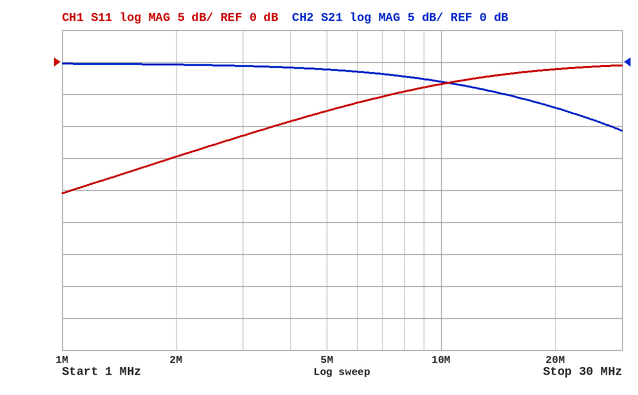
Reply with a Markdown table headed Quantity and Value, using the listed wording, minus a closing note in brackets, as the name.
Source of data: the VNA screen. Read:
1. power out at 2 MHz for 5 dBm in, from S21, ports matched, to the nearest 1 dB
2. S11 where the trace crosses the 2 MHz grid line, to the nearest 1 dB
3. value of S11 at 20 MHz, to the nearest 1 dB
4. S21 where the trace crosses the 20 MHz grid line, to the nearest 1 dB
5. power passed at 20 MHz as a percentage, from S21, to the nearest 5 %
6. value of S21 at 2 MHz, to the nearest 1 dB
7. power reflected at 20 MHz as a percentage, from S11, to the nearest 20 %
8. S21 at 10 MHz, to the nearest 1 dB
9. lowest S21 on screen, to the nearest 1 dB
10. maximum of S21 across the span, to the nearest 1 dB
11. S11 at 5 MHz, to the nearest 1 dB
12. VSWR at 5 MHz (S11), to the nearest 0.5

| Quantity | Value |
|---|---|
| power out at 2 MHz for 5 dBm in, from S21, ports matched, to the nearest 1 dB | 5 dBm |
| S11 where the trace crosses the 2 MHz grid line, to the nearest 1 dB | -15 dB |
| value of S11 at 20 MHz, to the nearest 1 dB | -1 dB |
| S21 where the trace crosses the 20 MHz grid line, to the nearest 1 dB | -7 dB |
| power passed at 20 MHz as a percentage, from S21, to the nearest 5 % | 20 % |
| value of S21 at 2 MHz, to the nearest 1 dB | 0 dB |
| power reflected at 20 MHz as a percentage, from S11, to the nearest 20 % | 80 % |
| S21 at 10 MHz, to the nearest 1 dB | -3 dB |
| lowest S21 on screen, to the nearest 1 dB | -11 dB |
| maximum of S21 across the span, to the nearest 1 dB | 0 dB |
| S11 at 5 MHz, to the nearest 1 dB | -8 dB |
| VSWR at 5 MHz (S11), to the nearest 0.5 | 2.5 |
